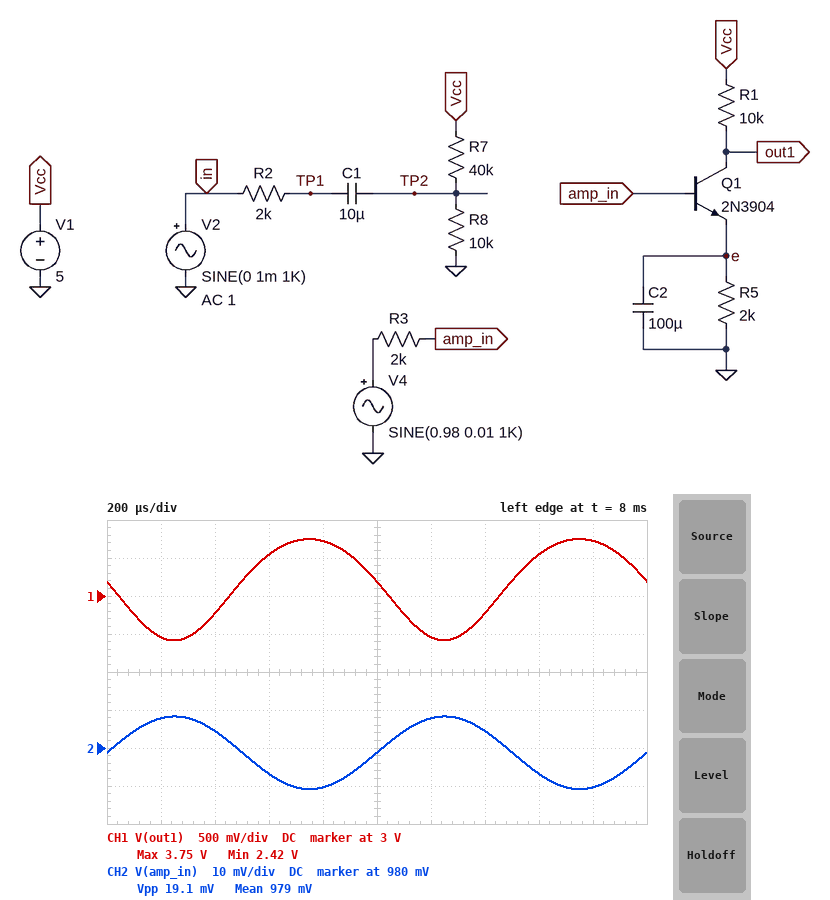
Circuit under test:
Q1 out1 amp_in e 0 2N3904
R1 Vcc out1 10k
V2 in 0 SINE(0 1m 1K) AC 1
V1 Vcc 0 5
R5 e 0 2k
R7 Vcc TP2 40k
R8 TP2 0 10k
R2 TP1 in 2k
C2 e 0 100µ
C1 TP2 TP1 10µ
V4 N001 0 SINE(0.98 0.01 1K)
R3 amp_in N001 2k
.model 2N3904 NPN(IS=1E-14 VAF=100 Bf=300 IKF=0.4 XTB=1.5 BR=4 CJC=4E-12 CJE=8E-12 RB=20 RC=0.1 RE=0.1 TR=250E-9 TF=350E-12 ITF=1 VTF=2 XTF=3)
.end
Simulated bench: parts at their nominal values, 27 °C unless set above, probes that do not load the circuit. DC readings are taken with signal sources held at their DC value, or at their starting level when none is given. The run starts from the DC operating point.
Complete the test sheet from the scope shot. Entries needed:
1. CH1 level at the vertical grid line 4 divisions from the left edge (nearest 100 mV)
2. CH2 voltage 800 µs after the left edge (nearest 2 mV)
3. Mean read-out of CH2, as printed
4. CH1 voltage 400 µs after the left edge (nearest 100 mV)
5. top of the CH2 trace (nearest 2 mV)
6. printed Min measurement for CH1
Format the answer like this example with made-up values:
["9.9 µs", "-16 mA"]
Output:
["3.7 V", "970 mV", "979 mV", "2.8 V", "988 mV", "2.42 V"]
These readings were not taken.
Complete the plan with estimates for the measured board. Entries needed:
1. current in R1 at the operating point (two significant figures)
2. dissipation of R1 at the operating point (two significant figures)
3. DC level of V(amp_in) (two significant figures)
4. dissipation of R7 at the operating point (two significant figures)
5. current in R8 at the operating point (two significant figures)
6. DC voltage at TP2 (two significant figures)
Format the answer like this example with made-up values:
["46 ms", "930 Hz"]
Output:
["180 µA", "340 µW", "980 mV", "400 µW", "100 µA", "1.0 V"]
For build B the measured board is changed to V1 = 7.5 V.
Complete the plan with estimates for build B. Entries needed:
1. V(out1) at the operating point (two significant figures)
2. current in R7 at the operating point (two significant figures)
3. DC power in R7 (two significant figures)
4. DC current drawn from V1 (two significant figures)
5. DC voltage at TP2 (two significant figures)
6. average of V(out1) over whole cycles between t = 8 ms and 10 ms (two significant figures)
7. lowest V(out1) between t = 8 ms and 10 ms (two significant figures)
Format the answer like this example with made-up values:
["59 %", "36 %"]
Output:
["5.7 V", "150 µA", "900 µW", "330 µA", "1.5 V", "5.6 V", "4.9 V"]
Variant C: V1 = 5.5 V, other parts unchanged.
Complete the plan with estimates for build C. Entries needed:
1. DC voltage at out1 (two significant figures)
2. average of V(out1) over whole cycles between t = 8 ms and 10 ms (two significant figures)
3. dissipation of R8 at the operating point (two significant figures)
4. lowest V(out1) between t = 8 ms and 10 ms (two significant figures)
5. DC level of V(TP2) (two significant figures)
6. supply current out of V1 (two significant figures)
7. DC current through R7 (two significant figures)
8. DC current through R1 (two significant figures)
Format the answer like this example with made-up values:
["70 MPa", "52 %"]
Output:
["3.7 V", "3.6 V", "120 µW", "2.9 V", "1.1 V", "290 µA", "110 µA", "180 µA"]
